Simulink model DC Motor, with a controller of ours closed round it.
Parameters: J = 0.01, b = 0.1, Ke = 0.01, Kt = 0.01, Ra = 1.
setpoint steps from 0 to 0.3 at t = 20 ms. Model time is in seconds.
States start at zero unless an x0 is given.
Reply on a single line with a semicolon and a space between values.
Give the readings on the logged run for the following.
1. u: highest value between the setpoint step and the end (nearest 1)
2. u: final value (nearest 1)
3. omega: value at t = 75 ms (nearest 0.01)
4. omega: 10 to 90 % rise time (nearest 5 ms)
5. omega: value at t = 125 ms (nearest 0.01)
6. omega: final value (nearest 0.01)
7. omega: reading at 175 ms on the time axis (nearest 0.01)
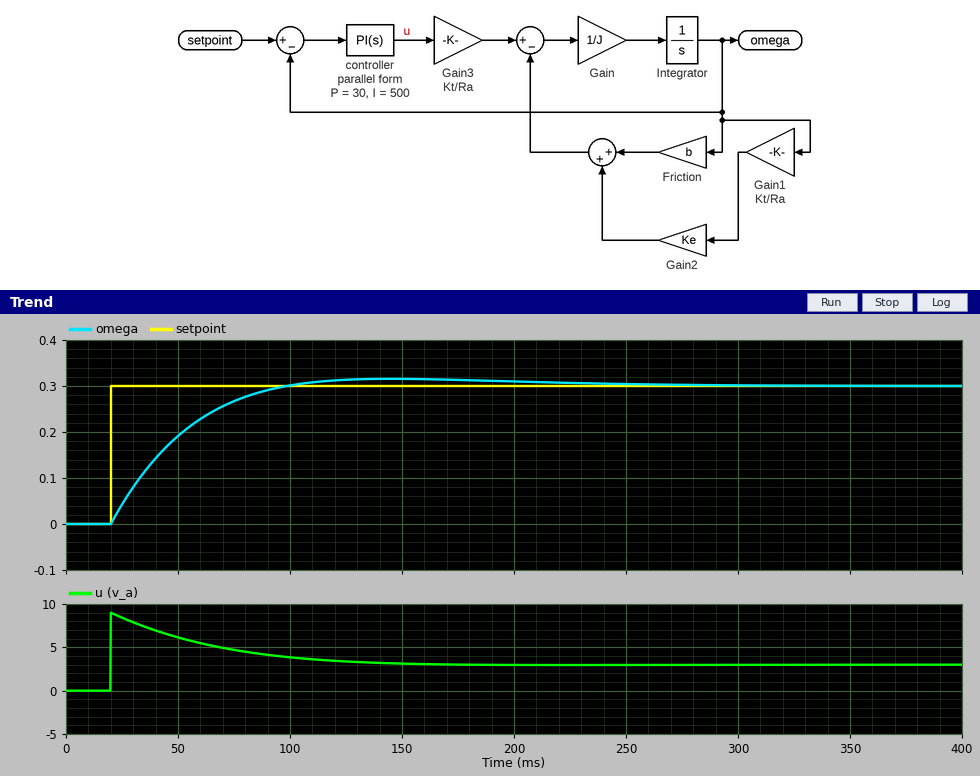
9; 3; 0.27; 55 ms; 0.31; 0.30; 0.31
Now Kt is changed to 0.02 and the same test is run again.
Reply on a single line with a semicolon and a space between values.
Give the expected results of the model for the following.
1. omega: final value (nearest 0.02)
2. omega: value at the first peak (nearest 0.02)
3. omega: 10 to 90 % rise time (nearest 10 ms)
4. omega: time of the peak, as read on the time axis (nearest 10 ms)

0.30; 0.32; 30 ms; 100 ms
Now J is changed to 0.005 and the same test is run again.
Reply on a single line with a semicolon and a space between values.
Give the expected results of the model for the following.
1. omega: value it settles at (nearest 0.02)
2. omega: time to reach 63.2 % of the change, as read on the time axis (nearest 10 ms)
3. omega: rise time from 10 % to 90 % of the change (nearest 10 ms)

0.30; 40 ms; 40 ms
